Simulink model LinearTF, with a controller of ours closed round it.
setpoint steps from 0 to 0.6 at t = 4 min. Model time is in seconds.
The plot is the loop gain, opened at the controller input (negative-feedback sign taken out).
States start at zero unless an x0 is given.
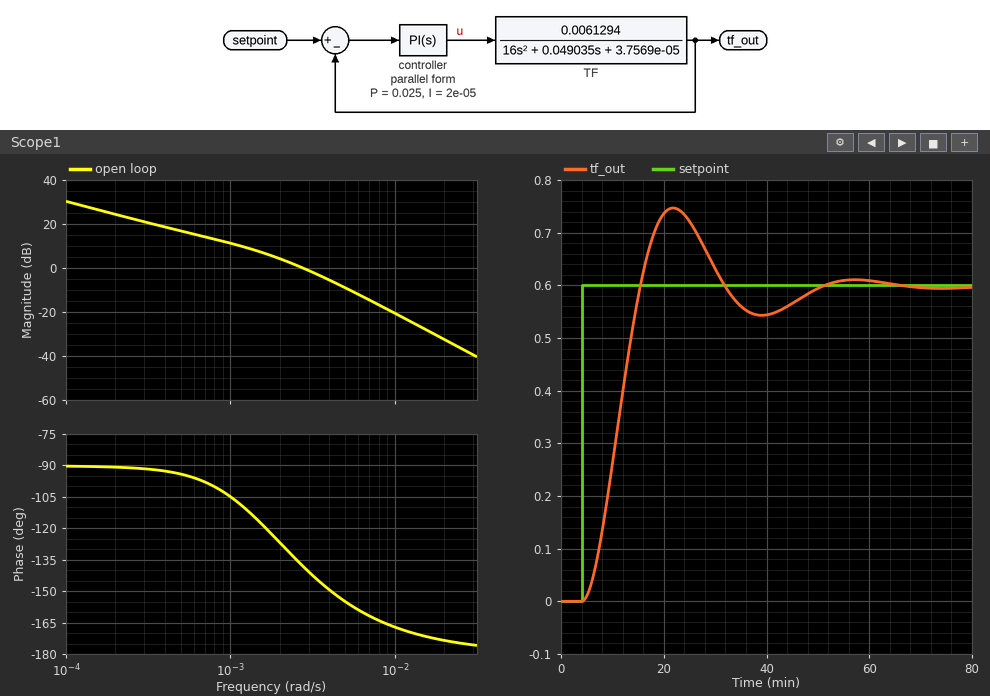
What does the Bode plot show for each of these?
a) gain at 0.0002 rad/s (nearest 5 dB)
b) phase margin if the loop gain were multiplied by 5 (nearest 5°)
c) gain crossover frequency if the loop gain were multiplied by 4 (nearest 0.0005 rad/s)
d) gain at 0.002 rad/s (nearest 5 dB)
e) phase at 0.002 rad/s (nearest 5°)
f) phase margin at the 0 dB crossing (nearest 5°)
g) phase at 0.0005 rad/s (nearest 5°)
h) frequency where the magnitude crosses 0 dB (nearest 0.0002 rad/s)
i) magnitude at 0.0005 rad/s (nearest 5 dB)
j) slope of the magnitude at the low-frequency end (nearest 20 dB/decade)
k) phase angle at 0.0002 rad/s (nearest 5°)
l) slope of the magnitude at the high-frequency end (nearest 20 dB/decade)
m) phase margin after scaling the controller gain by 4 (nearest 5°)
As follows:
25 dB
20°
0.0060 rad/s
5 dB
-125°
40°
-95°
0.0028 rad/s
15 dB
-20 dB/decade
-90°
-40 dB/decade
20°
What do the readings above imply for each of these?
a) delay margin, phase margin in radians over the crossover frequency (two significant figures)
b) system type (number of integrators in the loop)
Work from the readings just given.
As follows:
250 s
1
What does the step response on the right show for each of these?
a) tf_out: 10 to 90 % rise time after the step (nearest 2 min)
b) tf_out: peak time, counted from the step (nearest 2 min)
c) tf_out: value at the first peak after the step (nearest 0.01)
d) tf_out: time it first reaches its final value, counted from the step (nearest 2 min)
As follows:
8 min
18 min
0.75
12 min
